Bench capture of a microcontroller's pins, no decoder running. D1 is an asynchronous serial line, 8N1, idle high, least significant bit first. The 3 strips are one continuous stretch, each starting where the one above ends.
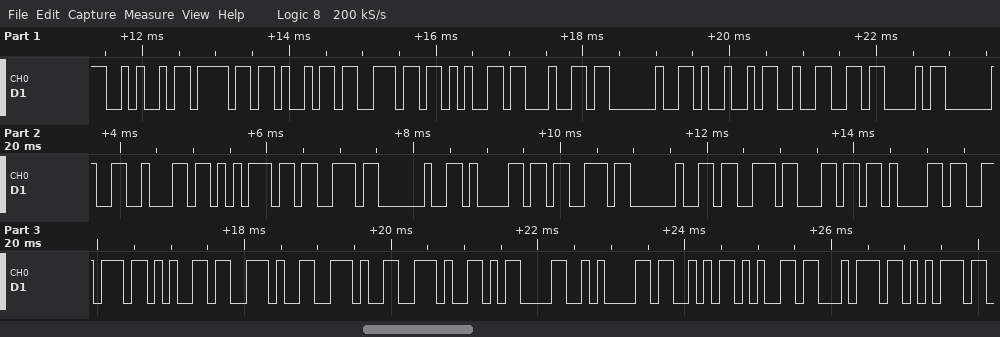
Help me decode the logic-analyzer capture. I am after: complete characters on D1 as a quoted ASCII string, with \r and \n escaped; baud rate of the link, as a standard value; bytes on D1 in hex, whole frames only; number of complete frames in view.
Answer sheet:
"Joined I2C bus as slave...\r\nSetu"
9600 baud
4A 6F 69 6E 65 64 20 49 32 43 20 62 75 73 20 61 73 20 73 6C 61 76 65 2E 2E 2E 0D 0A 53 65 74 75
32
